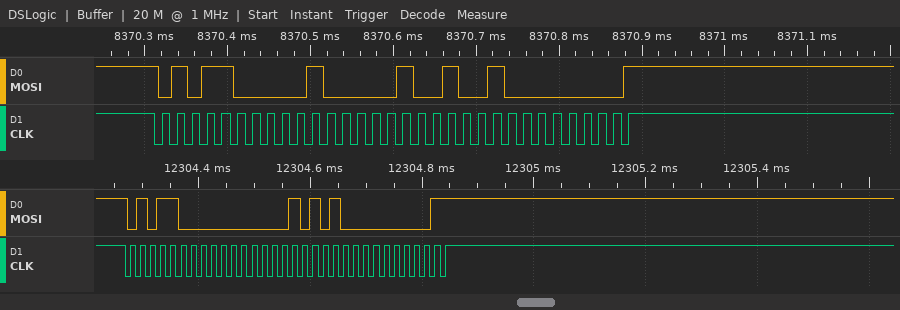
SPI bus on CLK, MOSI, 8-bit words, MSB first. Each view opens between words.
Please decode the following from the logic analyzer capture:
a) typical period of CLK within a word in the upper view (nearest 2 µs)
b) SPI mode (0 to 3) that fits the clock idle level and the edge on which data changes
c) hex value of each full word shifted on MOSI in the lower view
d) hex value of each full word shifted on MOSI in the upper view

18 µs
3
58, 00, A8, 03
58, 20, 92, 01
